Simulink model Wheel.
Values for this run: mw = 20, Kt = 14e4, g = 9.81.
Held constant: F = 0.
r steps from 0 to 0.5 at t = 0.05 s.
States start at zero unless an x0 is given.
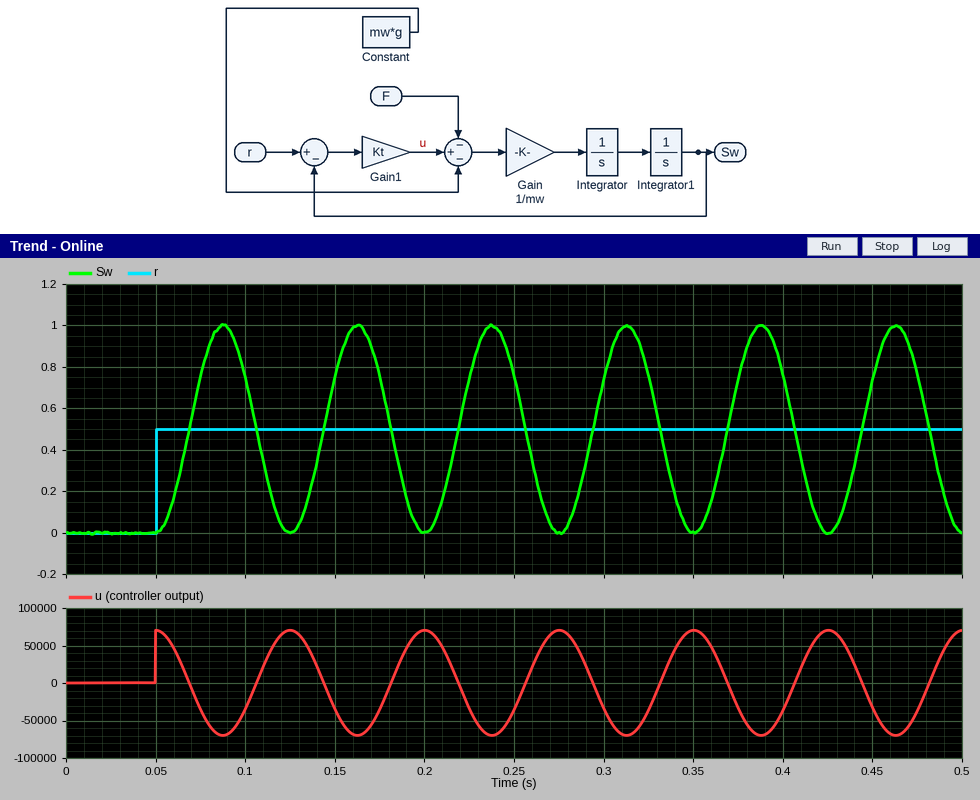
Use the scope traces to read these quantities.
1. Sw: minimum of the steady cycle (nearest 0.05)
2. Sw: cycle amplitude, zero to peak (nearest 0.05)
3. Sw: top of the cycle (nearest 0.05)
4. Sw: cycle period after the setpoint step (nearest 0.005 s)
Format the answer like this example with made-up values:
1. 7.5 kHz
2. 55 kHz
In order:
1. 0.00
2. 0.50
3. 1.00
4. 0.075 s
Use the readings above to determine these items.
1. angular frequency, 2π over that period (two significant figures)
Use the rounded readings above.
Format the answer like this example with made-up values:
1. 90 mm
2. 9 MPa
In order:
1. 84 rad/s
